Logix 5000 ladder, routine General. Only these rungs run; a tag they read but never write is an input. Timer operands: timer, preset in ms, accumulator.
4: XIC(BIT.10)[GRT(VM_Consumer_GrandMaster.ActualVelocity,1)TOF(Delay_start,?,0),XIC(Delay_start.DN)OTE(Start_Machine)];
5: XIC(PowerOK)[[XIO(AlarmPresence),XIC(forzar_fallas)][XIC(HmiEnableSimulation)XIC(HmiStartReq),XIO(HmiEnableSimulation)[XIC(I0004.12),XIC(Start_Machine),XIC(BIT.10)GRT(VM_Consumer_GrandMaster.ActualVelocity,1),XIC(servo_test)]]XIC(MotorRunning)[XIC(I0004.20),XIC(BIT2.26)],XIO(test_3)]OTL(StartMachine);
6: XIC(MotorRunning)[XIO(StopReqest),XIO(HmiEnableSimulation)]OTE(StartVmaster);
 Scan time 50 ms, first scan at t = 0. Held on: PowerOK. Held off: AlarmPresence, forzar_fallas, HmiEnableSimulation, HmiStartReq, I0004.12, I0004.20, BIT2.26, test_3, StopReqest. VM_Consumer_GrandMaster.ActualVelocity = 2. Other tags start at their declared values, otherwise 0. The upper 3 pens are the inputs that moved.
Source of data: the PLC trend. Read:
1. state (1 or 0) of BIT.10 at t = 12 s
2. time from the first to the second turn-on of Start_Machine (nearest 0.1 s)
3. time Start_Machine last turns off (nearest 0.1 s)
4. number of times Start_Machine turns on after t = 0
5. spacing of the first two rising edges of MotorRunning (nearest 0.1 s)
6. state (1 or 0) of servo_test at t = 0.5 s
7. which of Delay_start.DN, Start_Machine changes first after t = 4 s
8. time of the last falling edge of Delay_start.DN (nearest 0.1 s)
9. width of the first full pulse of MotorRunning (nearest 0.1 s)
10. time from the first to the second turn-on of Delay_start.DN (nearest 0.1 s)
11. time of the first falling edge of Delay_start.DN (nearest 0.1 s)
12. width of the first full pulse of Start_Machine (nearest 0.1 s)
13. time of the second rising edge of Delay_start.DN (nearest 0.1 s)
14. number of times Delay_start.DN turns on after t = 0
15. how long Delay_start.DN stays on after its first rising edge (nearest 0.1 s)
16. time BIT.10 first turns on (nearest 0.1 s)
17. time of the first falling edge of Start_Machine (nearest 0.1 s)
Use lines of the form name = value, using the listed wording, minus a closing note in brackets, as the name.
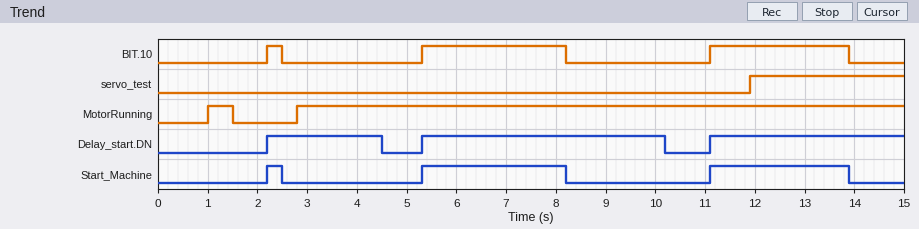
state (1 or 0) of BIT.10 at t = 12 s = 1
time from the first to the second turn-on of Start_Machine = 3.1 s
time Start_Machine last turns off = 13.9 s
number of times Start_Machine turns on after t = 0 = 3
spacing of the first two rising edges of MotorRunning = 1.8 s
state (1 or 0) of servo_test at t = 0.5 s = 0
which of Delay_start.DN, Start_Machine changes first after t = 4 s = Delay_start.DN
time of the last falling edge of Delay_start.DN = 10.2 s
width of the first full pulse of MotorRunning = 0.5 s
time from the first to the second turn-on of Delay_start.DN = 3.1 s
time of the first falling edge of Delay_start.DN = 4.5 s
width of the first full pulse of Start_Machine = 0.3 s
time of the second rising edge of Delay_start.DN = 5.3 s
number of times Delay_start.DN turns on after t = 0 = 3
how long Delay_start.DN stays on after its first rising edge = 2.3 s
time BIT.10 first turns on = 2.2 s
time of the first falling edge of Start_Machine = 2.5 s
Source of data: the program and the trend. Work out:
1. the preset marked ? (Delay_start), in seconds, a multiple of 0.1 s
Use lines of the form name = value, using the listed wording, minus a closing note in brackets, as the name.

the preset marked ? (Delay_start), in seconds, a multiple of 0.1 s = 2.0 s
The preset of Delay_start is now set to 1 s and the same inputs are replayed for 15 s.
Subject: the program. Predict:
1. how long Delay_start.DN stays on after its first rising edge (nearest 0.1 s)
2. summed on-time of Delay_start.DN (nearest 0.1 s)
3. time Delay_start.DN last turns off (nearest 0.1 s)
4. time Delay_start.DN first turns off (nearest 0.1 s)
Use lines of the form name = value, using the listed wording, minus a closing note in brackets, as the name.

how long Delay_start.DN stays on after its first rising edge = 1.3 s
summed on-time of Delay_start.DN = 9.0 s
time Delay_start.DN last turns off = 14.9 s
time Delay_start.DN first turns off = 3.5 s
